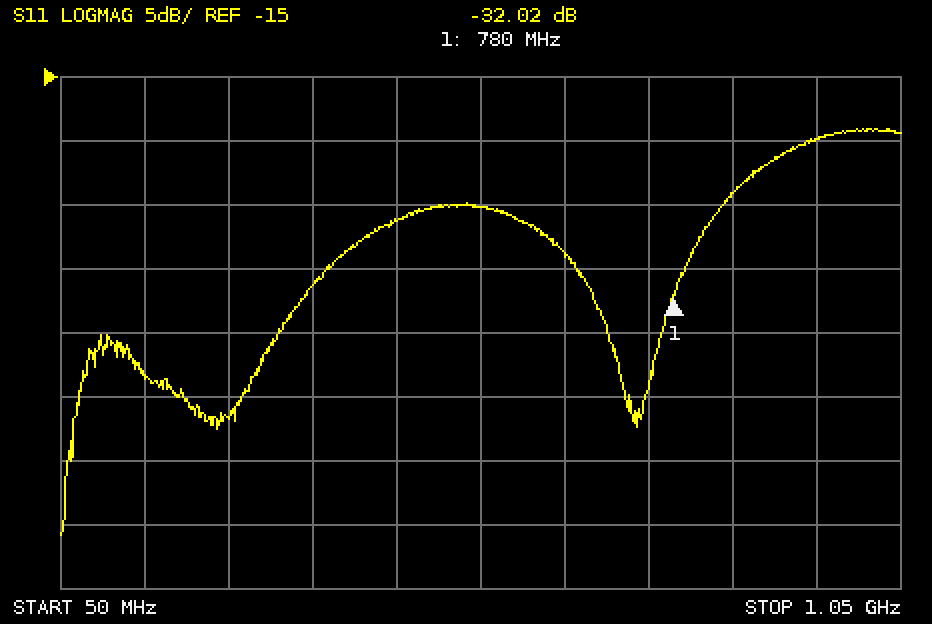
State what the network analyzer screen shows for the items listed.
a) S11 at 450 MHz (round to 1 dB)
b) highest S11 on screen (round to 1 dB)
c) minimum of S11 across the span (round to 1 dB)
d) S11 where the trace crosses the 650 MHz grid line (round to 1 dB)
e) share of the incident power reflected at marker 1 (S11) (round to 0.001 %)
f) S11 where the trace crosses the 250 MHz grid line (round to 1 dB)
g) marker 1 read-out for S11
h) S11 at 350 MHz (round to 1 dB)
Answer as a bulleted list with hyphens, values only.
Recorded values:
- -26 dB
- -19 dB
- -51 dB
- -29 dB
- 0.063 %
- -42 dB
- -32.02 dB
- -31 dB
